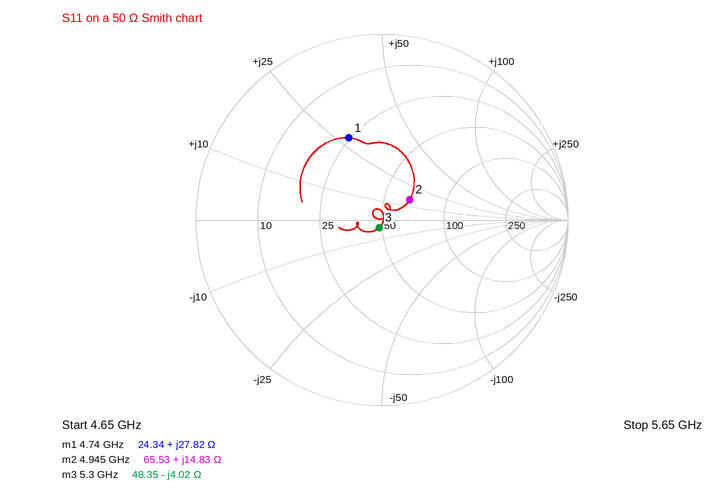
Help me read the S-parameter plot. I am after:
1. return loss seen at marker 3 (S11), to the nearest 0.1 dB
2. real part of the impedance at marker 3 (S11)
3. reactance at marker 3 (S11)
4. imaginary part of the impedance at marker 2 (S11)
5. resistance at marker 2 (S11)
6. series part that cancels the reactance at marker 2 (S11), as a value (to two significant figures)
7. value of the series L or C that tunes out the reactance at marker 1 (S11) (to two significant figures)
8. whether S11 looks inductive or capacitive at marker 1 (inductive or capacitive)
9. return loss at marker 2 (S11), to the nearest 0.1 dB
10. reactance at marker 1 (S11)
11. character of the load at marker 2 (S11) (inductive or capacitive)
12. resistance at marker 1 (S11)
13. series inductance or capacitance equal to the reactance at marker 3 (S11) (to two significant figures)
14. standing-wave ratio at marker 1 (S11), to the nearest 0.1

27.1 dB
48.35 Ω
-4.02 Ω
+14.83 Ω
65.53 Ω
2.2 pF
1.2 pF
inductive
14.7 dB
+27.82 Ω
inductive
24.34 Ω
7.5 pF
2.8
